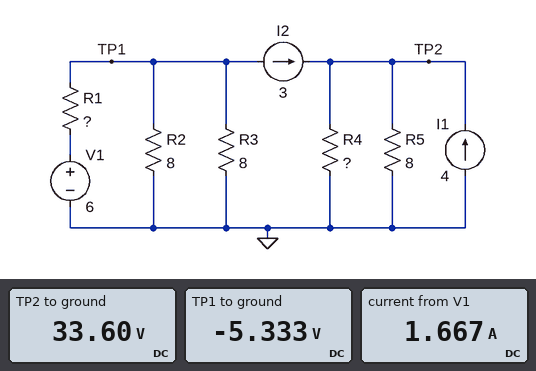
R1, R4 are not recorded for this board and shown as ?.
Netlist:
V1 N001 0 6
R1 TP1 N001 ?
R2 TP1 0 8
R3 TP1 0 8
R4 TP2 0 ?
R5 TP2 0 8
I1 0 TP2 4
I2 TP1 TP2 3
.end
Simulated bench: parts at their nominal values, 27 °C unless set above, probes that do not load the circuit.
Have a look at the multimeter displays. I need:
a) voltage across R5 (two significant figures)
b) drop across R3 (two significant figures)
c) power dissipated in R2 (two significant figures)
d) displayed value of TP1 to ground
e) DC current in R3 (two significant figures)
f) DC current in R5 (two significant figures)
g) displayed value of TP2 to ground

34 V
5.3 V
3.6 W
-5.333 V
670 mA
4.2 A
33.60 V
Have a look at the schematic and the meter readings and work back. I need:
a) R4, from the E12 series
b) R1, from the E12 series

12 Ω
6.8 Ω
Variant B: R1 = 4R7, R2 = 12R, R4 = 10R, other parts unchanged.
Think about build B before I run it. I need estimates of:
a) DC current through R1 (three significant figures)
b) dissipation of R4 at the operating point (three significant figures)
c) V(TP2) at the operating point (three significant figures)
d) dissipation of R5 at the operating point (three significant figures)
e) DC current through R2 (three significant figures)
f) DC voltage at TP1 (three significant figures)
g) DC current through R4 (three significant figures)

2.15 A
96.8 W
31.1 V
121 W
341 mA
-4.09 V
3.11 A
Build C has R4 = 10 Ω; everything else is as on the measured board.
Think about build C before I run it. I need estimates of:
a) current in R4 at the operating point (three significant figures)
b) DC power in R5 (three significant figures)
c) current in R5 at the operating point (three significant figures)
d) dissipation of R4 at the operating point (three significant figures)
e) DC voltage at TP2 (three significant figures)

3.11 A
121 W
3.89 A
96.8 W
31.1 V
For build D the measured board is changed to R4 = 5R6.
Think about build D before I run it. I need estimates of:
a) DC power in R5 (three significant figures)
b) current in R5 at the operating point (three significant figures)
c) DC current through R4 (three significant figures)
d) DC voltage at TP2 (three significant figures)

66.5 W
2.88 A
4.12 A
23.1 V
